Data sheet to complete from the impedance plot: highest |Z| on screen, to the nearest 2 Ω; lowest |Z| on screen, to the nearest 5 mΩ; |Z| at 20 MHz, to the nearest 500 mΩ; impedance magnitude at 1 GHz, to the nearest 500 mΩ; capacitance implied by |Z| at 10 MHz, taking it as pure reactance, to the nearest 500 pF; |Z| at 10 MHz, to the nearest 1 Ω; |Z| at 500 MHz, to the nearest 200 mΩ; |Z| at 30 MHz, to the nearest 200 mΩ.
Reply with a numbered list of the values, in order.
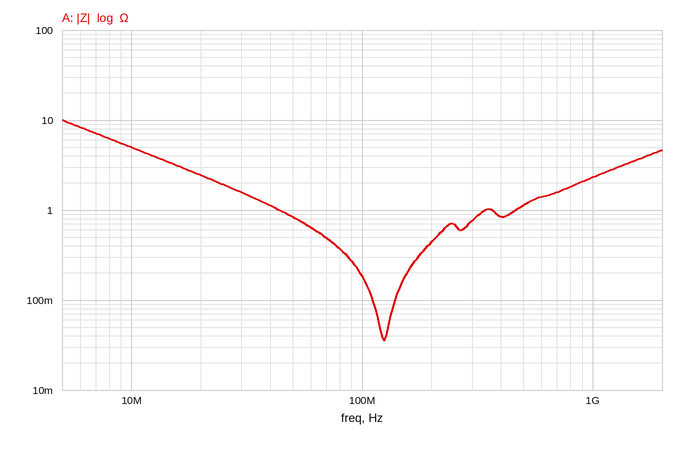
1. 10 Ω
2. 35 mΩ
3. 2.5 Ω
4. 2.5 Ω
5. 3.0 nF
6. 5 Ω
7. 1.2 Ω
8. 1.6 Ω
